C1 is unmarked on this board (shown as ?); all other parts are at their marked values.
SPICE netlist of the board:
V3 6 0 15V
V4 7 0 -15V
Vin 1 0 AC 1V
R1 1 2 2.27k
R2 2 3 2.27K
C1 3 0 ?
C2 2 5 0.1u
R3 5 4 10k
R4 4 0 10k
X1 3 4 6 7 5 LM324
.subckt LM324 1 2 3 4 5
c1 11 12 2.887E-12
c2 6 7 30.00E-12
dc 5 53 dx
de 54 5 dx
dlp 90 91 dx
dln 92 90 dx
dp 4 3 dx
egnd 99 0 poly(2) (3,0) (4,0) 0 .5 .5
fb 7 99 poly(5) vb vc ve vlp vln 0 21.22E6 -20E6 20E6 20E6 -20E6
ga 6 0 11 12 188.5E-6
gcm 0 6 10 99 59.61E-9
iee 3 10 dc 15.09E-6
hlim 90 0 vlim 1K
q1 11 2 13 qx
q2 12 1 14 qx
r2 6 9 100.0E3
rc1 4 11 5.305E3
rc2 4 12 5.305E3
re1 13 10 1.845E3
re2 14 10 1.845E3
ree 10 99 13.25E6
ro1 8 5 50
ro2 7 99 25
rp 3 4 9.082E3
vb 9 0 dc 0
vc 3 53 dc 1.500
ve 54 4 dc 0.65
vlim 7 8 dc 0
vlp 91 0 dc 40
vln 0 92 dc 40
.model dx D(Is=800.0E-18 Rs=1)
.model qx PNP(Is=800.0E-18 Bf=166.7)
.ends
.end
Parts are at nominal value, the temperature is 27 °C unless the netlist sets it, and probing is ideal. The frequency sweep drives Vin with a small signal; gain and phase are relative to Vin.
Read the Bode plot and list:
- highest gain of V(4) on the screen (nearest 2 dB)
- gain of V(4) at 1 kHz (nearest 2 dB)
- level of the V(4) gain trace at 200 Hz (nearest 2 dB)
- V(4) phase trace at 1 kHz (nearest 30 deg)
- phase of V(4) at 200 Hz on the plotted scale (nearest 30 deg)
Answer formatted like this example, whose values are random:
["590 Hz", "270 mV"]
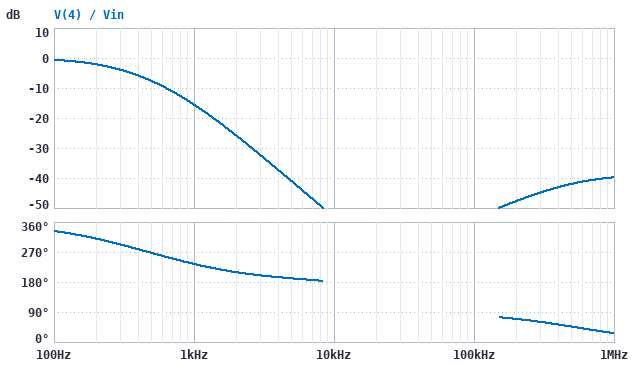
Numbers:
["0 dB", "-16 dB", "-2 dB", "240 deg", "300 deg"]
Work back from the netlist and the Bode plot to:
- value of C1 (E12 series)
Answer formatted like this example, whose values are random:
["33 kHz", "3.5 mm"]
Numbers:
["220 nF"]
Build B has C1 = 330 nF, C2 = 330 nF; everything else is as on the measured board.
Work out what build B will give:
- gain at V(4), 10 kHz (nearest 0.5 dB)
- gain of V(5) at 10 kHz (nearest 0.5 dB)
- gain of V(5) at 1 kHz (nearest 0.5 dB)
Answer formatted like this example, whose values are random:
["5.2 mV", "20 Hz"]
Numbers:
["-66.0 dB", "-60.0 dB", "-20.5 dB"]
